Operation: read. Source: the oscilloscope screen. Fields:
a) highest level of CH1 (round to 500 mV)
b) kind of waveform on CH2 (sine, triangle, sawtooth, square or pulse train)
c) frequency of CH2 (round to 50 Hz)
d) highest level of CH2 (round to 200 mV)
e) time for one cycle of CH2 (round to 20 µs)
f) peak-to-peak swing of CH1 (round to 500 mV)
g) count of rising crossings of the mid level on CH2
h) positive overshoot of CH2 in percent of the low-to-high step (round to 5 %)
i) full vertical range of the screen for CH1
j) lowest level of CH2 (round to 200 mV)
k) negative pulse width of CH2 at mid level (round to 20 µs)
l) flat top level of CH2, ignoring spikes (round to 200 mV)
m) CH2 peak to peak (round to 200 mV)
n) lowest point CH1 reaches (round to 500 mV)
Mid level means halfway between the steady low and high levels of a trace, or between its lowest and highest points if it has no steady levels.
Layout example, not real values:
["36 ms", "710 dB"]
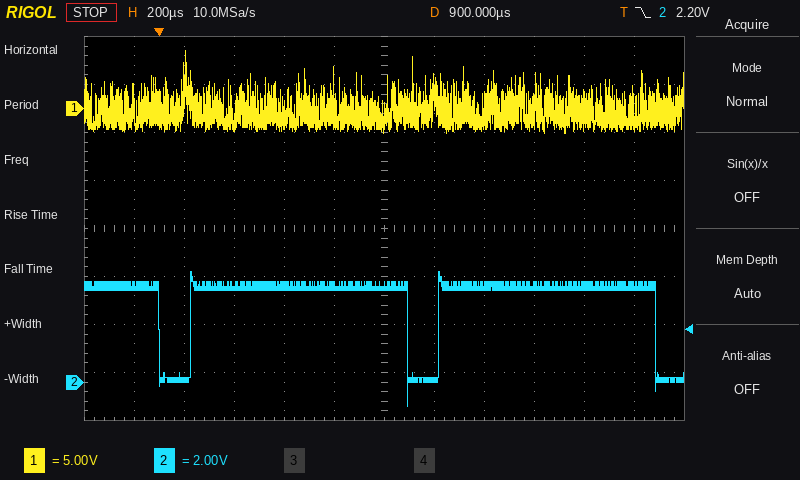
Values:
["6.0 V", "pulse train", "1.00 kHz", "4.6 V", "1.00 ms", "8.5 V", "2", "15 %", "40 V", "-1.0 V", "120 µs", "4.0 V", "5.6 V", "-2.5 V"]
